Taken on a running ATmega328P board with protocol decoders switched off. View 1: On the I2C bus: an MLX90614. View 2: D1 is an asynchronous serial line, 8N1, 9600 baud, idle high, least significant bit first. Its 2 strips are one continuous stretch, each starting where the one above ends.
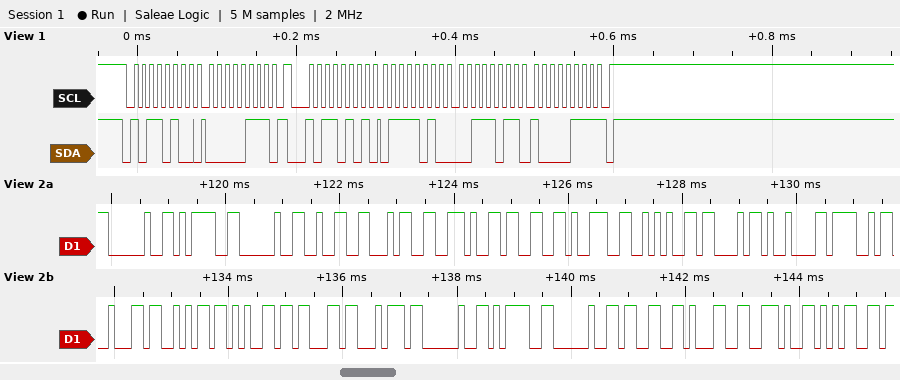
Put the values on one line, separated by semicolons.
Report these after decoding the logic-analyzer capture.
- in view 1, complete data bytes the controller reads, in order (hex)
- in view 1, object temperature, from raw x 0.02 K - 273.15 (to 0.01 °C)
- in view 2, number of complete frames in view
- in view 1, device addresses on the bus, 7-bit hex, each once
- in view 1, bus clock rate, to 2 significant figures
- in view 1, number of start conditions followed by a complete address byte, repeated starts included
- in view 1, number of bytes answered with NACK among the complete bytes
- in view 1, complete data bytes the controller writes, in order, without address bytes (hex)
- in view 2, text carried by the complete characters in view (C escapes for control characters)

7A 3B 87; 31.37 °C; 24; 0x5A; 100 kHz; 2; 1; 07; " = 24.39*C\tObject = 31.5"
